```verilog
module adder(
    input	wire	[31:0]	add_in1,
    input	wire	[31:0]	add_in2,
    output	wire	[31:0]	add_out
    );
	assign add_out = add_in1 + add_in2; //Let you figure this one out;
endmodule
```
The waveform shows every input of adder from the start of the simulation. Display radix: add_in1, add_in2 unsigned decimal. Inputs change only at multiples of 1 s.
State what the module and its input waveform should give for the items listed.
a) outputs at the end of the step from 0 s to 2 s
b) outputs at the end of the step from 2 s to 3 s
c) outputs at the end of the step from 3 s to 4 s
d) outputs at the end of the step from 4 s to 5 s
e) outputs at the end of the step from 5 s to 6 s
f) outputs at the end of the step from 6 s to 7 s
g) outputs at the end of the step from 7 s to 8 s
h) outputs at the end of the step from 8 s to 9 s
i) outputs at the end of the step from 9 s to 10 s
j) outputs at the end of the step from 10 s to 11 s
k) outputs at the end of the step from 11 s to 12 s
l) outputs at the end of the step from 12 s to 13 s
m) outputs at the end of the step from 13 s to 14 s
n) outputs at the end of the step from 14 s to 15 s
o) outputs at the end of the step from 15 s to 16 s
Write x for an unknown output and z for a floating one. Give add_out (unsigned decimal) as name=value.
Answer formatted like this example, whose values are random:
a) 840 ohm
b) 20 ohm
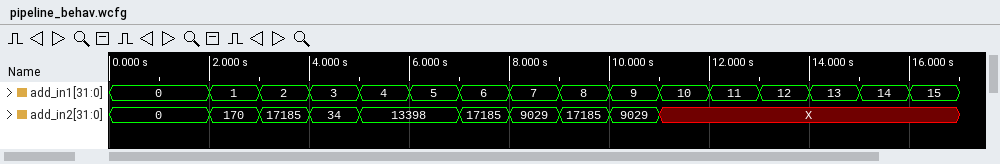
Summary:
a) add_out=0
b) add_out=171
c) add_out=17187
d) add_out=37
e) add_out=13402
f) add_out=13403
g) add_out=17191
h) add_out=9036
i) add_out=17193
j) add_out=9038
k) add_out=x
l) add_out=x
m) add_out=x
n) add_out=x
o) add_out=x
